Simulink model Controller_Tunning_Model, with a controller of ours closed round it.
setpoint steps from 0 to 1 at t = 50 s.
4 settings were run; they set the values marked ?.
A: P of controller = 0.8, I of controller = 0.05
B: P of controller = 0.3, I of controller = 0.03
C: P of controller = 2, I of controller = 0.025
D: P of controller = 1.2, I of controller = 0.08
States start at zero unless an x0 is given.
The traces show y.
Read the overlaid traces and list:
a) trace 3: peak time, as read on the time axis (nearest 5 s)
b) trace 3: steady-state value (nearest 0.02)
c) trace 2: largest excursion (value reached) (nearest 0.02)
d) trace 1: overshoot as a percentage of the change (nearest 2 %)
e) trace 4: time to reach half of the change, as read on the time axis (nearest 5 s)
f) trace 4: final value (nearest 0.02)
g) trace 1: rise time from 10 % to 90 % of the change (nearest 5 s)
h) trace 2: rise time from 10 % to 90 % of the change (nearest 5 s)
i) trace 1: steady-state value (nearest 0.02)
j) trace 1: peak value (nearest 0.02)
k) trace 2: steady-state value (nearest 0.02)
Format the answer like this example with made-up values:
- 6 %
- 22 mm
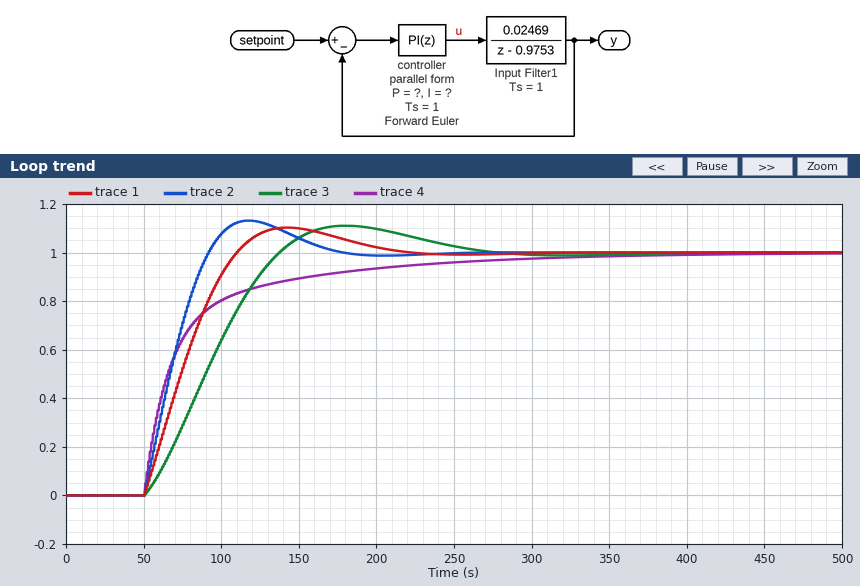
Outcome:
- 180 s
- 1.00
- 1.14
- 10 %
- 65 s
- 1.00
- 45 s
- 30 s
- 1.00
- 1.10
- 1.00
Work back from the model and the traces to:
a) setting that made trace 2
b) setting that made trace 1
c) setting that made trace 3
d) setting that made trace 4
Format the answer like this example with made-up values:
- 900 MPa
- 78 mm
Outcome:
- D
- A
- B
- C
